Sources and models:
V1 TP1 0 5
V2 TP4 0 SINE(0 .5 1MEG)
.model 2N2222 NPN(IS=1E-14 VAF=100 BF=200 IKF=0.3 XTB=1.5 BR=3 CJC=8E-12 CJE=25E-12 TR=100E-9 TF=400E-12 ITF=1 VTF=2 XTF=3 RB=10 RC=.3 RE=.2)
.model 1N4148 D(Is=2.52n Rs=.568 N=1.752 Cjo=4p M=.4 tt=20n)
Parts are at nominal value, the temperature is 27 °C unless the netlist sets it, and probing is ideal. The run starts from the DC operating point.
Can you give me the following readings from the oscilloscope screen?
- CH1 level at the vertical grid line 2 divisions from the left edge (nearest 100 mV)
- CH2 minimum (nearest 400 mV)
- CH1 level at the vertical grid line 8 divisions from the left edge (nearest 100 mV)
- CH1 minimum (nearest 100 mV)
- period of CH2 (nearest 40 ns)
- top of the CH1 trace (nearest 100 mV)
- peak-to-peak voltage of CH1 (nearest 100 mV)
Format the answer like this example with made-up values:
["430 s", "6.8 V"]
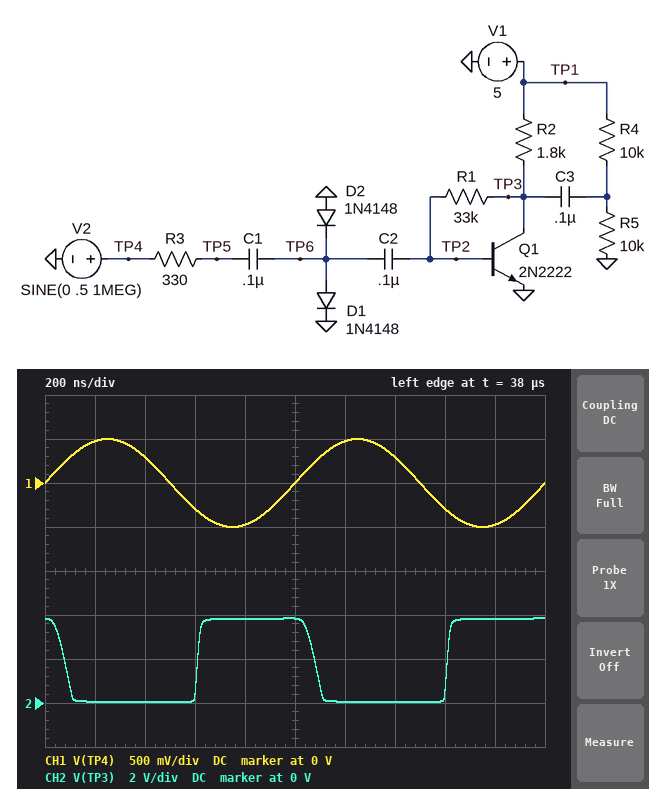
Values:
["300 mV", "0 V", "-300 mV", "-500 mV", "1.00 µs", "500 mV", "1.0 V"]
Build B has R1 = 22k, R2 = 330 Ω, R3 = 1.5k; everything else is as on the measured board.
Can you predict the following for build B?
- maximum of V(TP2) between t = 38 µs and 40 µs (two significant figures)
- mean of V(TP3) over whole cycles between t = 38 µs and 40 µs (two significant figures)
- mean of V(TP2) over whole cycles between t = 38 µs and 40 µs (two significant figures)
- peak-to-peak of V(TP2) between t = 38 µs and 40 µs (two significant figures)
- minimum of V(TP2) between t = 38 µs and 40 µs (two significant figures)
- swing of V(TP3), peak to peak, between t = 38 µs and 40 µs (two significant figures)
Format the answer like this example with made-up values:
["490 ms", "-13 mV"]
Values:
["730 mV", "2.0 V", "690 mV", "170 mV", "560 mV", "4.6 V"]
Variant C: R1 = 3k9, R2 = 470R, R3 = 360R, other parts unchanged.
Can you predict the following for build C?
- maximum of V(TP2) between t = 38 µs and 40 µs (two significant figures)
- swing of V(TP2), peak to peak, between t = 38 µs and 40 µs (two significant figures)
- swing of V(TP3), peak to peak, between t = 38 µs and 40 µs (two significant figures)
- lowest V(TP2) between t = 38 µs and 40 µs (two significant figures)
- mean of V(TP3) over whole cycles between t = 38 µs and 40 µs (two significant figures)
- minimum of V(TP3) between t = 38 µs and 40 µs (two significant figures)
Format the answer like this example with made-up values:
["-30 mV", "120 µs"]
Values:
["740 mV", "200 mV", "4.2 V", "530 mV", "1.5 V", "61 mV"]
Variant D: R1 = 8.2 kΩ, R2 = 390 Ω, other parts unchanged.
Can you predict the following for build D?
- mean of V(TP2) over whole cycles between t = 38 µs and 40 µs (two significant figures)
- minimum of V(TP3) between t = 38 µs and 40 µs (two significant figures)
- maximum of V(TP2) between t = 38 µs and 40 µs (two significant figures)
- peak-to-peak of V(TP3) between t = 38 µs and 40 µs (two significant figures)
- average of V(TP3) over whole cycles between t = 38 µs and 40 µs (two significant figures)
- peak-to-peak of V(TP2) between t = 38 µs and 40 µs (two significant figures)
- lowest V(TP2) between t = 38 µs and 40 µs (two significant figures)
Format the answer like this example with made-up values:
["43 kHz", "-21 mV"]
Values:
["620 mV", "66 mV", "740 mV", "4.5 V", "1.9 V", "430 mV", "310 mV"]
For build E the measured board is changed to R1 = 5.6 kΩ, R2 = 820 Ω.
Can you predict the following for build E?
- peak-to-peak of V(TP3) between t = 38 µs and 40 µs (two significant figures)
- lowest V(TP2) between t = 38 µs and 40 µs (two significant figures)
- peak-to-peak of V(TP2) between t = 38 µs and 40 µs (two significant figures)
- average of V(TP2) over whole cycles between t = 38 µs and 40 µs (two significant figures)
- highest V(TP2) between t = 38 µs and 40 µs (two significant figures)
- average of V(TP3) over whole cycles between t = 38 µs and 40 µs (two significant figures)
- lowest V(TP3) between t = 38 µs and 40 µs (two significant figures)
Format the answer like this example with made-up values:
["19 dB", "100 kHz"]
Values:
["3.9 V", "350 mV", "370 mV", "620 mV", "720 mV", "1.6 V", "46 mV"]
